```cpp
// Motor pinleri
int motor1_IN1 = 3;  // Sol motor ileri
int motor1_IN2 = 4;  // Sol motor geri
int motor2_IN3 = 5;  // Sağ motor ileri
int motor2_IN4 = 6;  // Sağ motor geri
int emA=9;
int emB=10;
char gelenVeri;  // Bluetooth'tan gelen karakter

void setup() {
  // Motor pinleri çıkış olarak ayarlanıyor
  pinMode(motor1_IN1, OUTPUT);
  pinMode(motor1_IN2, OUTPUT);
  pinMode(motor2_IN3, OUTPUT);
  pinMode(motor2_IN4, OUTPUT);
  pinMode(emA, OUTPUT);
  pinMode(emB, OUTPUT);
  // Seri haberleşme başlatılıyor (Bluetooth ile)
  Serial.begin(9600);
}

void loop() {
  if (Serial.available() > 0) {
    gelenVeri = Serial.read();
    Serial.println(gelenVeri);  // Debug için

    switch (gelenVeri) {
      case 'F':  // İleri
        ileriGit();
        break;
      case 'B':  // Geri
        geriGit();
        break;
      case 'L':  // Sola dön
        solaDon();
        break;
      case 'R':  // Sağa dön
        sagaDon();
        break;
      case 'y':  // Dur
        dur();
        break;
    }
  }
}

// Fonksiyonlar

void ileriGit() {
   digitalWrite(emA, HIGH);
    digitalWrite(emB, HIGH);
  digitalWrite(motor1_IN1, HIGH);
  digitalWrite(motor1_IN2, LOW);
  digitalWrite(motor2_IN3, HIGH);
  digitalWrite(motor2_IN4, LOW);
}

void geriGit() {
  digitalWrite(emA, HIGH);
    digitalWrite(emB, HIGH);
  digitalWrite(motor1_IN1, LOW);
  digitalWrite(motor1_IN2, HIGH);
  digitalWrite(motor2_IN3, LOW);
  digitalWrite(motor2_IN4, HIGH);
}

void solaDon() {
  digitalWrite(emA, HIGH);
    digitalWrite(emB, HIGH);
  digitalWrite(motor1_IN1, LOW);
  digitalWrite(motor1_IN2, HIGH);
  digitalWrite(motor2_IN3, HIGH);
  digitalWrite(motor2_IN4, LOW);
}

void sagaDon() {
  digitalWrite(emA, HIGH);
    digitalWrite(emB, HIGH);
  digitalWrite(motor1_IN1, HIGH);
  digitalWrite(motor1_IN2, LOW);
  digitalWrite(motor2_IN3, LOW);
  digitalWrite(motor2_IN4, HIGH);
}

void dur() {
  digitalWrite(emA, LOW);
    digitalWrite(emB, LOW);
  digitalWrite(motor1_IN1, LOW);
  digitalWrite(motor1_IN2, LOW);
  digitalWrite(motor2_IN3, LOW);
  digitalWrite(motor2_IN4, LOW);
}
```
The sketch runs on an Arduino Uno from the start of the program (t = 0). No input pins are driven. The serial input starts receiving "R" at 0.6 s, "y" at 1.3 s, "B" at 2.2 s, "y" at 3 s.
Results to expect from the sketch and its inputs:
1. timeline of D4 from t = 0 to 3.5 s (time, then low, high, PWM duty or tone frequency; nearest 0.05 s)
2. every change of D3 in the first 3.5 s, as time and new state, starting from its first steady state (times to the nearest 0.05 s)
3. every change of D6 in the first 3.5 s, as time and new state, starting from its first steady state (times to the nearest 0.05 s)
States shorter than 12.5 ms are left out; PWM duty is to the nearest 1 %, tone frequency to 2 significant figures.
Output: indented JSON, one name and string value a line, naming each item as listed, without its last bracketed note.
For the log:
{
  "timeline of D4 from t = 0 to 3.5 s": "0 s low; 2.2 s high; 3 s low",
  "every change of D3 in the first 3.5 s, as time and new state, starting from its first steady state": "0 s low; 0.6 s high; 1.3 s low",
  "every change of D6 in the first 3.5 s, as time and new state, starting from its first steady state": "0 s low; 0.6 s high; 1.3 s low; 2.2 s high; 3 s low"
}
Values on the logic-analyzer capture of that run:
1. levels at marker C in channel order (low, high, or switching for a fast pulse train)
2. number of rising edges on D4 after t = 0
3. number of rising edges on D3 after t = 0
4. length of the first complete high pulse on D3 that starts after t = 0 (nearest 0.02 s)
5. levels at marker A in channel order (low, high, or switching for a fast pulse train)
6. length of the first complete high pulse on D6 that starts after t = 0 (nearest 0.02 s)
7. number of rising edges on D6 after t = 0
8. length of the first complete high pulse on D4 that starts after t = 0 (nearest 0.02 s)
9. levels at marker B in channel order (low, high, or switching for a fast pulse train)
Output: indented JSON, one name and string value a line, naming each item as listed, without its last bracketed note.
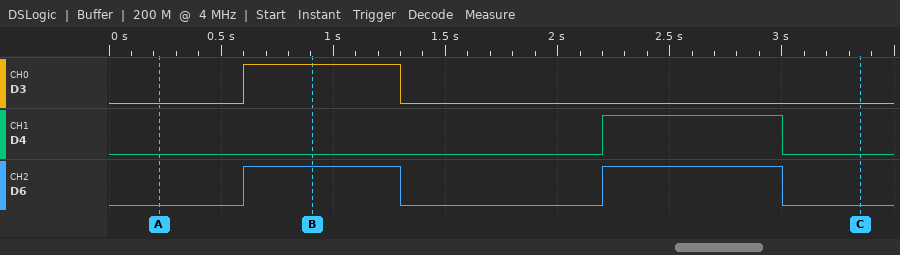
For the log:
{
  "levels at marker C in channel order": "D3 low, D4 low, D6 low",
  "number of rising edges on D4 after t = 0": "1",
  "number of rising edges on D3 after t = 0": "1",
  "length of the first complete high pulse on D3 that starts after t = 0": "0.70 s",
  "levels at marker A in channel order": "D3 low, D4 low, D6 low",
  "length of the first complete high pulse on D6 that starts after t = 0": "0.70 s",
  "number of rising edges on D6 after t = 0": "2",
  "length of the first complete high pulse on D4 that starts after t = 0": "0.80 s",
  "levels at marker B in channel order": "D3 high, D4 low, D6 high"
}
